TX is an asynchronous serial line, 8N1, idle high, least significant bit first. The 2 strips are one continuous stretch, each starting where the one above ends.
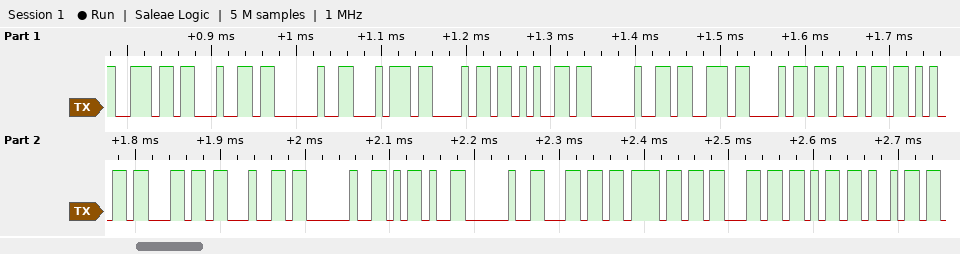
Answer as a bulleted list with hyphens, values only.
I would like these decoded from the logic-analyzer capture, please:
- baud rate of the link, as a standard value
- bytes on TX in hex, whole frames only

- 115200 baud
- 6E 64 20 74 68 65 20 73 68 69 65 6C 64 20 2D 20 6C 6F 63 6B 69
